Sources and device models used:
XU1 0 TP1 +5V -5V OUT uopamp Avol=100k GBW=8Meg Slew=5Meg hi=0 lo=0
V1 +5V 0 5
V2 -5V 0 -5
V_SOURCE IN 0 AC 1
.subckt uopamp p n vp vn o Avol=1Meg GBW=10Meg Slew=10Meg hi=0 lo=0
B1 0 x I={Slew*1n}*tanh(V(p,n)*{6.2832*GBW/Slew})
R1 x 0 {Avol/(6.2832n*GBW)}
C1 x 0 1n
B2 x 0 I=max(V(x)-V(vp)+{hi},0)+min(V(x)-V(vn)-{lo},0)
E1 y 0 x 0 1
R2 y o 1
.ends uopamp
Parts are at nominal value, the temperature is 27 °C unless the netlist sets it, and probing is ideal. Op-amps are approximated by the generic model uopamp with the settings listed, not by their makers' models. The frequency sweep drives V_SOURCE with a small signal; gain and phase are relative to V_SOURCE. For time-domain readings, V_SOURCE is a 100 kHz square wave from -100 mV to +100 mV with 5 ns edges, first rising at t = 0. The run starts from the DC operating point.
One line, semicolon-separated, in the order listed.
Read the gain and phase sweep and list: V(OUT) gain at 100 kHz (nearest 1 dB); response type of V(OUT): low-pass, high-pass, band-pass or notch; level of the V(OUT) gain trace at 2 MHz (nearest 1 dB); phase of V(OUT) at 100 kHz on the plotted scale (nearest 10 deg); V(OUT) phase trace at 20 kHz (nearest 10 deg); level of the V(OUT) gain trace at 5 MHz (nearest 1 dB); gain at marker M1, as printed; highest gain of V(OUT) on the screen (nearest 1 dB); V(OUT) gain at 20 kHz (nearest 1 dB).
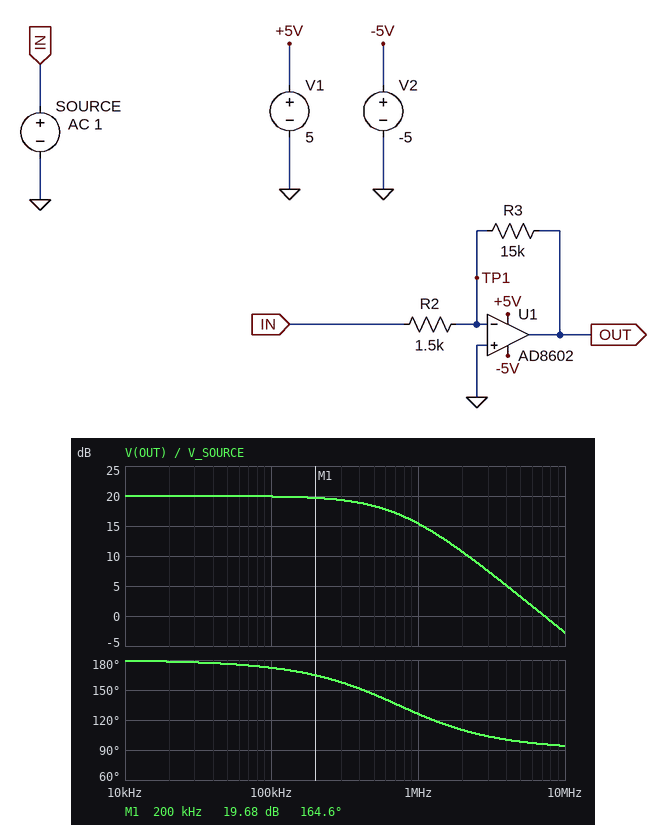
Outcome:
20 dB; low-pass; 11 dB; 170 deg; 180 deg; 3 dB; 19.68 dB; 20 dB; 20 dB
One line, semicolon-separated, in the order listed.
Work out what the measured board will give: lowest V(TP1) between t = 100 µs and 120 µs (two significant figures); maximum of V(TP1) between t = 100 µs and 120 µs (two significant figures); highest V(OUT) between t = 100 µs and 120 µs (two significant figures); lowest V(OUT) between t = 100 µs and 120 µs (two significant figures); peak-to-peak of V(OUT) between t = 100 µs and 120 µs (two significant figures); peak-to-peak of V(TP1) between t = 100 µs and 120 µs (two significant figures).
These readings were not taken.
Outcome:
-180 mV; 180 mV; 1.0 V; -1.0 V; 2.0 V; 360 mV
